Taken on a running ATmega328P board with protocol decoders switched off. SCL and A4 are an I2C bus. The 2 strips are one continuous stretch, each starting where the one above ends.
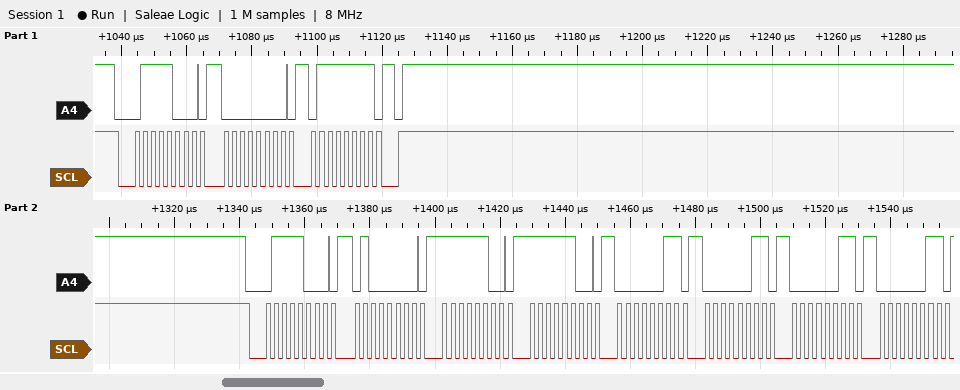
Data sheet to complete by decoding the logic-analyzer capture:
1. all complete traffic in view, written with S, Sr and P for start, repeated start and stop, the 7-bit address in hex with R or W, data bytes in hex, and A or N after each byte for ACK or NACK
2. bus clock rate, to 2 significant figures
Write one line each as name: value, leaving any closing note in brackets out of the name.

all complete traffic in view, written with S, Sr and P for start, repeated start and stop, the 7-bit address in hex with R or W, data bytes in hex, and A or N after each byte for ACK or NACK: S 3CW A 00 A 7F A P S 3CW A 40 A FC A FC A 03 A 03 A 03 A 03 A
bus clock rate, to 2 significant figures: 400 kHz
